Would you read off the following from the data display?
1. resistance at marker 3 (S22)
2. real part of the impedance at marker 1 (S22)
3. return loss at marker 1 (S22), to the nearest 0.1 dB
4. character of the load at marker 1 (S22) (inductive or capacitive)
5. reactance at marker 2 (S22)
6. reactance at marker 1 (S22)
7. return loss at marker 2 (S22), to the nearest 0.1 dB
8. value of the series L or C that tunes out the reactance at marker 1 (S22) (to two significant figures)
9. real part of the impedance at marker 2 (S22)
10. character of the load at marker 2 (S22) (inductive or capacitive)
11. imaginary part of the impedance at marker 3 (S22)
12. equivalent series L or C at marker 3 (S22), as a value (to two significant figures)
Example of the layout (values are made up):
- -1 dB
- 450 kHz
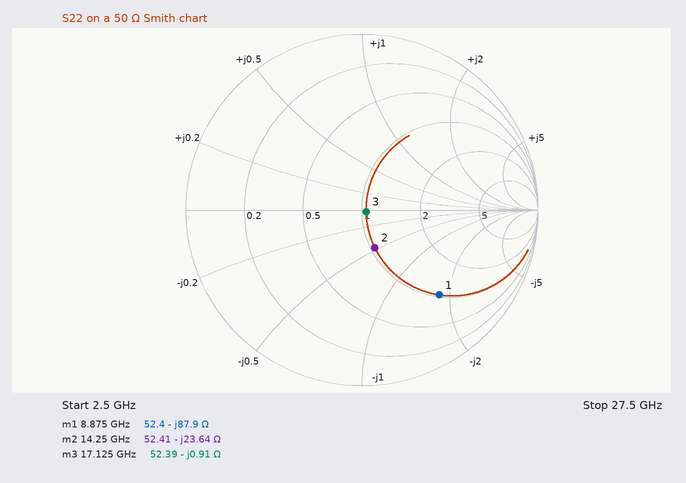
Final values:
- 52.39 Ω
- 52.4 Ω
- 3.7 dB
- capacitive
- -23.64 Ω
- -87.9 Ω
- 12.9 dB
- 1.6 nH
- 52.41 Ω
- capacitive
- -0.91 Ω
- 10 pF
